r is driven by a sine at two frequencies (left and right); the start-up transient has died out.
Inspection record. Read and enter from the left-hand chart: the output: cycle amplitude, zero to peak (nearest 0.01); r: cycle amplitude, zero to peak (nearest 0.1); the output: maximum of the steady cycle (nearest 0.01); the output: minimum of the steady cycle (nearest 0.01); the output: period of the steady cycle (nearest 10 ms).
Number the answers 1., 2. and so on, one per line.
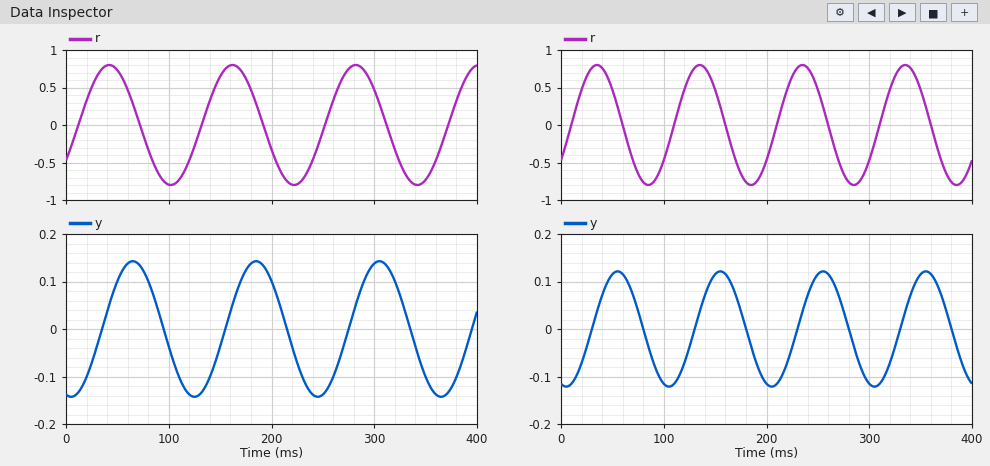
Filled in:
1. 0.14
2. 0.8
3. 0.14
4. -0.14
5. 120 ms
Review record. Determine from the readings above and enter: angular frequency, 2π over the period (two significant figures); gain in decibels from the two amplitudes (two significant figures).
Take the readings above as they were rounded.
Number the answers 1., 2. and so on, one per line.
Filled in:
1. 0.052 rad/ms
2. -15 dB
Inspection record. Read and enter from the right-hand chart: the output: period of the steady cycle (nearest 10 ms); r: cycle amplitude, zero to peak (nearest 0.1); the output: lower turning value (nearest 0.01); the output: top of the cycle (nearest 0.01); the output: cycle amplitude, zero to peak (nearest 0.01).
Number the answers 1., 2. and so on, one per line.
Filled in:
1. 100 ms
2. 0.8
3. -0.12
4. 0.12
5. 0.12
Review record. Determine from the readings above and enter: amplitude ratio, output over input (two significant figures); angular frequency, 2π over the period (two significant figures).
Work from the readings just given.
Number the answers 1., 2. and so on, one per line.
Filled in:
1. 0.15
2. 0.063 rad/ms
